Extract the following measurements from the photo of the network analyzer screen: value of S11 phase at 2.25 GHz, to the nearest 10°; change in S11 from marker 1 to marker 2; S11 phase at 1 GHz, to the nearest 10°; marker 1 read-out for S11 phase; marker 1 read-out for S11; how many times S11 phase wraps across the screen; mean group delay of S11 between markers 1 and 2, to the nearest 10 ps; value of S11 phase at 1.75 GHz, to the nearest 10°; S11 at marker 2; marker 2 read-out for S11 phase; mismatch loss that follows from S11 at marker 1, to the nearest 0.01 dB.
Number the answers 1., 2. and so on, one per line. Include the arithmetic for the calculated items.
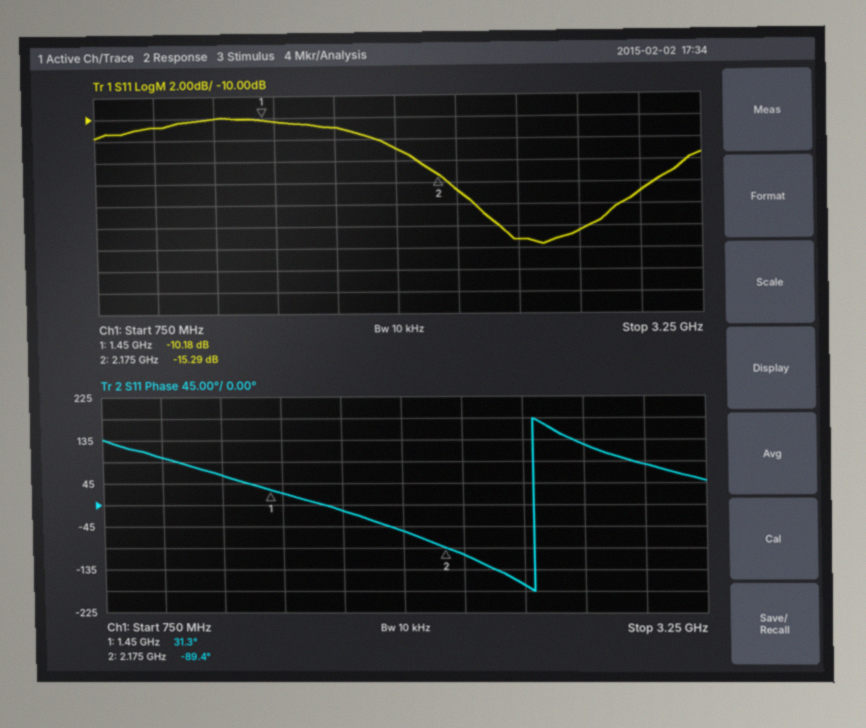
1. -100°
2. -15.29 − (-10.18) = -5.11 dB
3. 100°
4. 31.3°
5. -10.18 dB
6. 1
7. −(-89.4° − (31.3°))/(360° × 725 MHz) ≈ 462 ps, so 460 ps to the nearest 10 ps
8. -10°
9. -15.29 dB
10. -89.4°
11. −10 log10(1 − 10^(-10.18/10)) ≈ 0.44 dB
